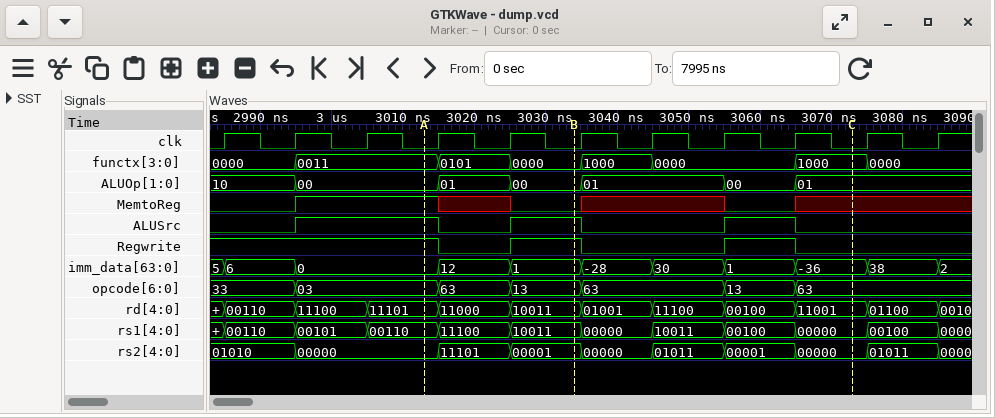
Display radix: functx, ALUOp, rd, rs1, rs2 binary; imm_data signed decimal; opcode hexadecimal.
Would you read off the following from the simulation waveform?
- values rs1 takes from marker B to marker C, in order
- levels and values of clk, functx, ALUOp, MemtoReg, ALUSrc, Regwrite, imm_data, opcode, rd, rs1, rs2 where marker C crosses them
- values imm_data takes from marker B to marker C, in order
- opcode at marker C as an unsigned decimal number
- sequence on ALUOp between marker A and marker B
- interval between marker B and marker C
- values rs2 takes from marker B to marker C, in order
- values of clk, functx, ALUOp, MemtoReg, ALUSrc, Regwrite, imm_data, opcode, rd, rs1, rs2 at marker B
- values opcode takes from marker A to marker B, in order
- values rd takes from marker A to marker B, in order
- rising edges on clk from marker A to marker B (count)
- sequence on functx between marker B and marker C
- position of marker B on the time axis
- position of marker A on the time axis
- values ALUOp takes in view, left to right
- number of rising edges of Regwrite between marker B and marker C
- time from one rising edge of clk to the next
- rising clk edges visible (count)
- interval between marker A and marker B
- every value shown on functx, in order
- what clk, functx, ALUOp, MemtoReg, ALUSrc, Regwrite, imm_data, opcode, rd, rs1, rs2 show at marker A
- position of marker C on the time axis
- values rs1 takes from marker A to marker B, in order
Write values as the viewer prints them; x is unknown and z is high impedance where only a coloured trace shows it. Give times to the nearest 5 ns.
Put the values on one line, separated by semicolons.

10011, 00000, 10011, 00100, 00000; clk=0, functx=1000, ALUOp=01, MemtoReg=x, ALUSrc=0, Regwrite=0, imm_data=-36, opcode=63, rd=11001, rs1=00000, rs2=00000; 1, -28, 30, 1, -36; 99; 00, 01, 00; 40 ns; 00001, 00000, 01011, 00001, 00000; clk=0, functx=0000, ALUOp=00, MemtoReg=0, ALUSrc=1, Regwrite=1, imm_data=1, opcode=13, rd=10011, rs1=10011, rs2=00001; 03, 63, 13; 11101, 11000, 10011; 2; 0000, 1000, 0000, 1000; 3035 ns; 3015 ns; 10, 00, 01, 00, 01, 00, 01; 1; 10 ns; 11; 20 ns; 0000, 0011, 0101, 0000, 1000, 0000, 1000, 0000; clk=0, functx=0011, ALUOp=00, MemtoReg=1, ALUSrc=1, Regwrite=1, imm_data=0, opcode=03, rd=11101, rs1=00110, rs2=00000; 3075 ns; 00110, 11100, 10011
